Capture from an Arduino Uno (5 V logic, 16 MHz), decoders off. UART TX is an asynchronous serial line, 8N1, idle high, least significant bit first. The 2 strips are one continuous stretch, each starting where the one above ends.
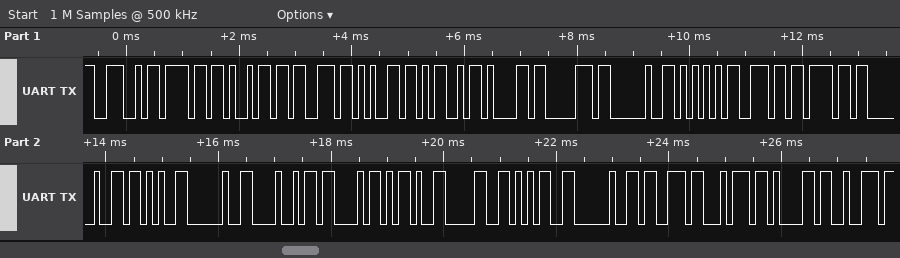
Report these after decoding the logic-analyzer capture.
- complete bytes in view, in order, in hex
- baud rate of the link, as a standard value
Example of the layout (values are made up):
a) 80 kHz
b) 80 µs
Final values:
a) 4E 6F 69 73 65 4D 61 70 20 55 6E 6F 20 2B 20 48 43 2D 30 35 20 73 74 61 72
b) 9600 baud
